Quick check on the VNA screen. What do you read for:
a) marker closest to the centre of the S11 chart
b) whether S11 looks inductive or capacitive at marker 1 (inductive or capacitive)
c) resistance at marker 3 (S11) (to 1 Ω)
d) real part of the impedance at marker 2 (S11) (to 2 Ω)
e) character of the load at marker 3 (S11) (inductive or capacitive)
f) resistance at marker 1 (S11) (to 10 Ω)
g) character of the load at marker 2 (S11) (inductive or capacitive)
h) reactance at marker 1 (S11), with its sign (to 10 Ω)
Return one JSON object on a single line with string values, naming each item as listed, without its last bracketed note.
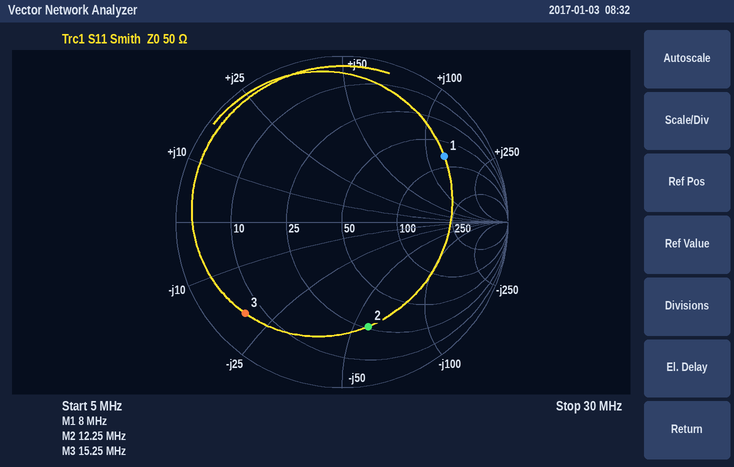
{"marker closest to the centre of the S11 chart": "marker 2", "whether S11 looks inductive or capacitive at marker 1": "inductive", "resistance at marker 3 (S11)": "6 Ω", "real part of the impedance at marker 2 (S11)": "26 Ω", "character of the load at marker 3 (S11)": "capacitive", "resistance at marker 1 (S11)": "80 Ω", "character of the load at marker 2 (S11)": "capacitive", "reactance at marker 1 (S11), with its sign": "+130 Ω"}
